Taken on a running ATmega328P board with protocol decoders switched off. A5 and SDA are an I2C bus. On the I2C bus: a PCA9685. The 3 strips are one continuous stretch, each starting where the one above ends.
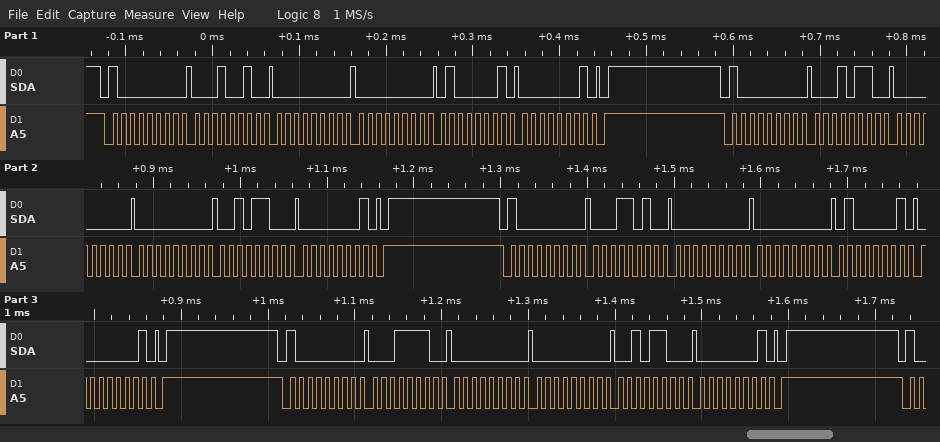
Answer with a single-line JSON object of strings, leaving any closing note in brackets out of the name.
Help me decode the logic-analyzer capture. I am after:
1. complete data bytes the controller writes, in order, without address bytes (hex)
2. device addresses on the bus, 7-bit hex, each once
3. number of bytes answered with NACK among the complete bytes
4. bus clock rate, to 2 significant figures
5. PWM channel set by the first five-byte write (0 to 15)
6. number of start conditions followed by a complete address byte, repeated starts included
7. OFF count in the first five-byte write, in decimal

{"complete data bytes the controller writes, in order, without address bytes": "12 00 00 41 01 16 00 00 2C 01 1A 00 00 41 01 1E 00 00 2C 01", "device addresses on the bus, 7-bit hex, each once": "0x40", "number of bytes answered with NACK among the complete bytes": "0", "bus clock rate, to 2 significant figures": "100 kHz", "PWM channel set by the first five-byte write": "3", "number of start conditions followed by a complete address byte, repeated starts included": "4", "OFF count in the first five-byte write, in decimal": "321"}
